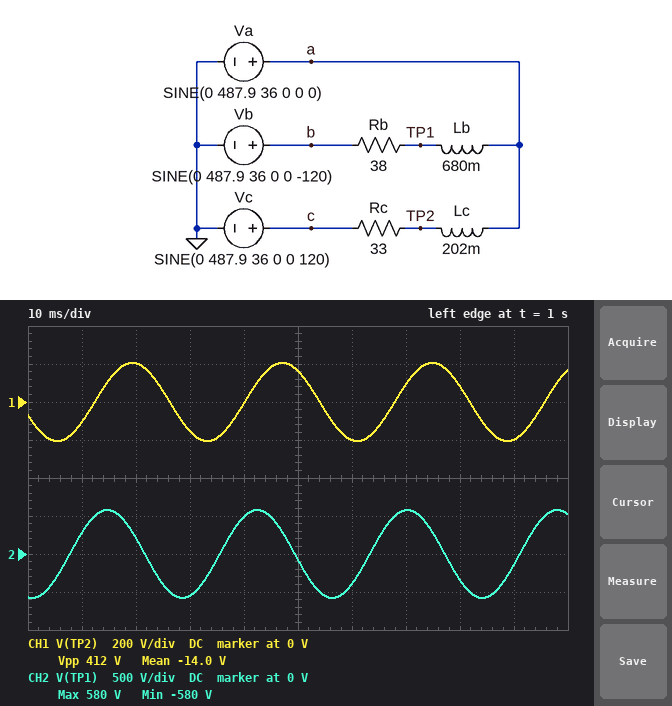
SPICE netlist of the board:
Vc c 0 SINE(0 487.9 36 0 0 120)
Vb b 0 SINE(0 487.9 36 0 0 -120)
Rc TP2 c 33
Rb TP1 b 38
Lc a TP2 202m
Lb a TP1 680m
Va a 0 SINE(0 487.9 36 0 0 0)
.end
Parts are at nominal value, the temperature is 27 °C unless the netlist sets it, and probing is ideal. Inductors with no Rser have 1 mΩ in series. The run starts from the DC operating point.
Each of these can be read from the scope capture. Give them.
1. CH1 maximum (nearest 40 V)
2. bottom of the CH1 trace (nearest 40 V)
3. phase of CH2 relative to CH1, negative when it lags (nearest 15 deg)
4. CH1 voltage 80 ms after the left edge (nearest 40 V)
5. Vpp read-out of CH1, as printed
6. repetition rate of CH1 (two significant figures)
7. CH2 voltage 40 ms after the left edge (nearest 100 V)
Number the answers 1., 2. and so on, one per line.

1. 200 V
2. -200 V
3. 60 deg
4. 80 V
5. 412 V
6. 36 Hz
7. 500 V
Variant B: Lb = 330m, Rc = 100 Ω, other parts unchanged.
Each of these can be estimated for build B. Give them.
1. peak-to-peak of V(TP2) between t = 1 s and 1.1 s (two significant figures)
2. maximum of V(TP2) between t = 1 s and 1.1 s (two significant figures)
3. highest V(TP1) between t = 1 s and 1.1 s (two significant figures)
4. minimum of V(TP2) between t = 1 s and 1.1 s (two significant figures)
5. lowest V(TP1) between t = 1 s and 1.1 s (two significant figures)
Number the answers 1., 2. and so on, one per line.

1. 570 V
2. 290 V
3. 640 V
4. -290 V
5. -640 V
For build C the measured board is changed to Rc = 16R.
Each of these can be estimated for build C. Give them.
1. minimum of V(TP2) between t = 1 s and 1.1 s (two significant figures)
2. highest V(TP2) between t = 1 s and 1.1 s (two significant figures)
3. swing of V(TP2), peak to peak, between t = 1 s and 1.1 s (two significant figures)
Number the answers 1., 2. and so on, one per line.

1. -330 V
2. 330 V
3. 660 V
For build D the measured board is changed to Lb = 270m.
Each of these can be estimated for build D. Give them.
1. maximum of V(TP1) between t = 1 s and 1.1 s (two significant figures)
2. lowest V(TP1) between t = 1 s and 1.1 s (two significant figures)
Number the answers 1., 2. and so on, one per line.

1. 650 V
2. -650 V
